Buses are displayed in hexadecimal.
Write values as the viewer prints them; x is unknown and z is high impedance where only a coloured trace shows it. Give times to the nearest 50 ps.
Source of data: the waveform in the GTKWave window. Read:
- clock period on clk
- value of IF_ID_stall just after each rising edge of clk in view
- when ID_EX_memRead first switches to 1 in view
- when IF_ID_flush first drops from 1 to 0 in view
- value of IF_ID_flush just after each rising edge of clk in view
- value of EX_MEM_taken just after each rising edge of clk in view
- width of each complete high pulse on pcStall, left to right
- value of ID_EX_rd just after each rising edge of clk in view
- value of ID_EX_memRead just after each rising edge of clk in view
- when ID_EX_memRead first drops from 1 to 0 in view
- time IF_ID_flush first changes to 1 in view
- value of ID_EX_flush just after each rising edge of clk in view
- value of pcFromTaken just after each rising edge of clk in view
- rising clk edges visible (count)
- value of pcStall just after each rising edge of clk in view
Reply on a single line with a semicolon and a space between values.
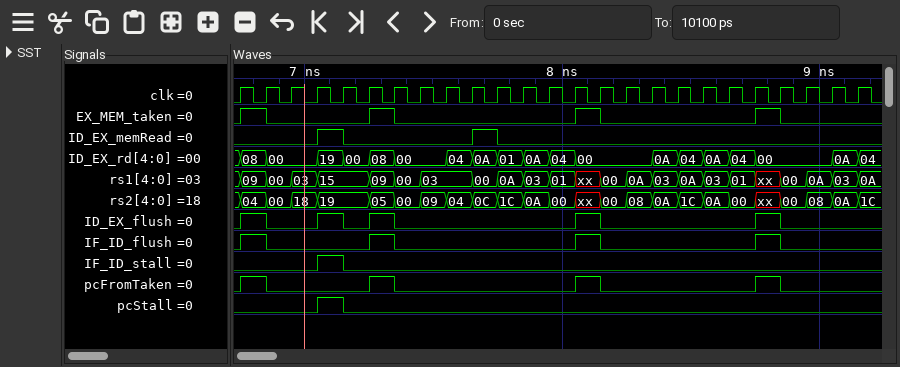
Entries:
100 ps; 0 0 0 1 0 0 0 0 0 0 0 0 0 0 0 0 0 0 0 0 0 0 0 0 0; 7050 ps; 6850 ps; 1 0 0 0 0 1 0 0 0 0 0 0 0 1 0 0 0 0 0 0 1 0 0 0 0; 1 0 0 0 0 1 0 0 0 0 0 0 0 1 0 0 0 0 0 0 1 0 0 0 0; 100 ps; 08, 00, 00, 19, 00, 08, 00, 00, 04, 0A, 01, 0A, 04, 00, 00, 00, 0A, 04, 0A, 04, 00, 00, 00, 0A, 04; 0 0 0 1 0 0 0 0 0 1 0 0 0 0 0 0 0 0 0 0 0 0 0 0 0; 7150 ps; 6750 ps; 1 0 0 1 0 1 0 0 0 0 0 0 0 1 0 0 0 0 0 0 1 0 0 0 0; 1 0 0 0 0 1 0 0 0 0 0 0 0 1 0 0 0 0 0 0 1 0 0 0 0; 25; 0 0 0 1 0 0 0 0 0 0 0 0 0 0 0 0 0 0 0 0 0 0 0 0 0
